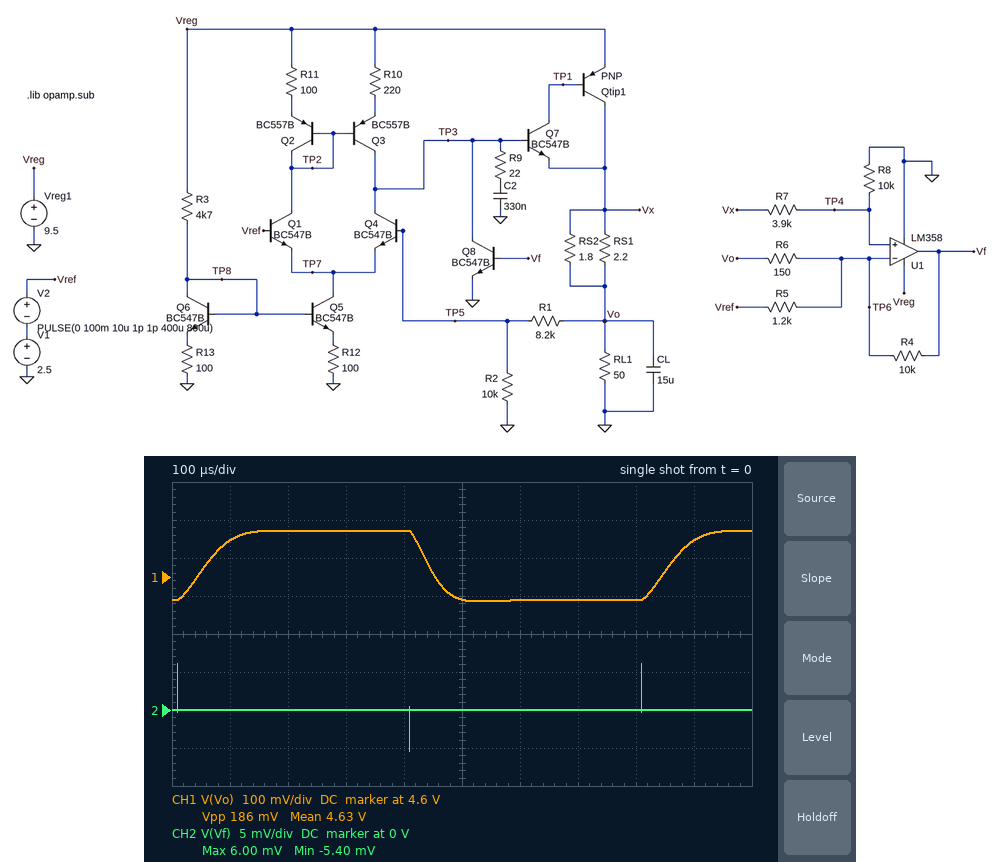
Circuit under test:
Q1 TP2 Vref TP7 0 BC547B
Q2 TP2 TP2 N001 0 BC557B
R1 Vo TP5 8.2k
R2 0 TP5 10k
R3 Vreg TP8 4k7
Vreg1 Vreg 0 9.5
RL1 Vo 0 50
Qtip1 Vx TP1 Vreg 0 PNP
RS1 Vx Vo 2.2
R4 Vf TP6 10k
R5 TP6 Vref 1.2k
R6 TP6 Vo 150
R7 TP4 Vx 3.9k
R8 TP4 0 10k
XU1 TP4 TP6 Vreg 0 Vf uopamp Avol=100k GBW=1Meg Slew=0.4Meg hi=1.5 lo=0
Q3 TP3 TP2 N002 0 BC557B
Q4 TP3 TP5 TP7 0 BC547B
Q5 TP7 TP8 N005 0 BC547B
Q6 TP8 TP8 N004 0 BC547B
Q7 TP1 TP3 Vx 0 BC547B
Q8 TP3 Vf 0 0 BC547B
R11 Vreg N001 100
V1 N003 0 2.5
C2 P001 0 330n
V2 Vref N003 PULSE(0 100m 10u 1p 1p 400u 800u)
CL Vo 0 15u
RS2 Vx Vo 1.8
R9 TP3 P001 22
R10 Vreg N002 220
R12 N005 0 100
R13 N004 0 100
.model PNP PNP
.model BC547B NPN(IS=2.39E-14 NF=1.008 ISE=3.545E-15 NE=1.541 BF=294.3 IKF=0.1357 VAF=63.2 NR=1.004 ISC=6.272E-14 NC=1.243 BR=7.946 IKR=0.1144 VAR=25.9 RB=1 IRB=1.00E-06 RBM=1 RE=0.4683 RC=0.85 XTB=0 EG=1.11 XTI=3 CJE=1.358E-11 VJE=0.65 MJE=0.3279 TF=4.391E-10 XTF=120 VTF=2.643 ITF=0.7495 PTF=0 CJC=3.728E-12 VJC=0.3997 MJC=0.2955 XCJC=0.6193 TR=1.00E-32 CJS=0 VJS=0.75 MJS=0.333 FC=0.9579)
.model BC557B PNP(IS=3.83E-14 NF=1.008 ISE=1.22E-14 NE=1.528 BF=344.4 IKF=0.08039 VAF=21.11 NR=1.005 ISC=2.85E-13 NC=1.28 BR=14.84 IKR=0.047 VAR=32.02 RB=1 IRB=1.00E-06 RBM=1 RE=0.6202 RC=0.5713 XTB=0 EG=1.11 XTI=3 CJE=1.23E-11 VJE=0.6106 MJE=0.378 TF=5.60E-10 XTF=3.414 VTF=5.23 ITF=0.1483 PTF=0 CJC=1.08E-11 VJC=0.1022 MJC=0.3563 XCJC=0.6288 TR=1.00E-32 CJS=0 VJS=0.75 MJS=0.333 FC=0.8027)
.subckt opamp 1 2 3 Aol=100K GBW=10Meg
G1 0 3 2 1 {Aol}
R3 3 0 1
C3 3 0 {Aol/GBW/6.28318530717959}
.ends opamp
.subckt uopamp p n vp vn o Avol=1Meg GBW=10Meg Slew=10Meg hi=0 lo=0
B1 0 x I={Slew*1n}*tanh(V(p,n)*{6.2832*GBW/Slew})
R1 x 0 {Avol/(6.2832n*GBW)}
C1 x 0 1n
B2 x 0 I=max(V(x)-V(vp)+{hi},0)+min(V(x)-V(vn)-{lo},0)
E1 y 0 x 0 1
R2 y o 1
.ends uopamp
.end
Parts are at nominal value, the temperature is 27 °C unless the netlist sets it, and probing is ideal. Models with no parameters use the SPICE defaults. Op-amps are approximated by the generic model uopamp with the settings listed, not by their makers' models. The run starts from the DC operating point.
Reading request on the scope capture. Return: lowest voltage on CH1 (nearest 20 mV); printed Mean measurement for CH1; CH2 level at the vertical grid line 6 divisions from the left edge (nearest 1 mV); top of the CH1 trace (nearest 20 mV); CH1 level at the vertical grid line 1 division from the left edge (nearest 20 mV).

4.54 V
4.63 V
0 V
4.72 V
4.70 V
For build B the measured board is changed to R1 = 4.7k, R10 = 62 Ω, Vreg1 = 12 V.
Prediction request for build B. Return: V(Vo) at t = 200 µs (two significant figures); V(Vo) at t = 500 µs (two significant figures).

3.9 V
3.7 V
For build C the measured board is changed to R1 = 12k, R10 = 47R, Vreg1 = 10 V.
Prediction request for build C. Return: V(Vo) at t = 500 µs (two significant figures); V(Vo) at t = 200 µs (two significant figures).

5.6 V
5.8 V
